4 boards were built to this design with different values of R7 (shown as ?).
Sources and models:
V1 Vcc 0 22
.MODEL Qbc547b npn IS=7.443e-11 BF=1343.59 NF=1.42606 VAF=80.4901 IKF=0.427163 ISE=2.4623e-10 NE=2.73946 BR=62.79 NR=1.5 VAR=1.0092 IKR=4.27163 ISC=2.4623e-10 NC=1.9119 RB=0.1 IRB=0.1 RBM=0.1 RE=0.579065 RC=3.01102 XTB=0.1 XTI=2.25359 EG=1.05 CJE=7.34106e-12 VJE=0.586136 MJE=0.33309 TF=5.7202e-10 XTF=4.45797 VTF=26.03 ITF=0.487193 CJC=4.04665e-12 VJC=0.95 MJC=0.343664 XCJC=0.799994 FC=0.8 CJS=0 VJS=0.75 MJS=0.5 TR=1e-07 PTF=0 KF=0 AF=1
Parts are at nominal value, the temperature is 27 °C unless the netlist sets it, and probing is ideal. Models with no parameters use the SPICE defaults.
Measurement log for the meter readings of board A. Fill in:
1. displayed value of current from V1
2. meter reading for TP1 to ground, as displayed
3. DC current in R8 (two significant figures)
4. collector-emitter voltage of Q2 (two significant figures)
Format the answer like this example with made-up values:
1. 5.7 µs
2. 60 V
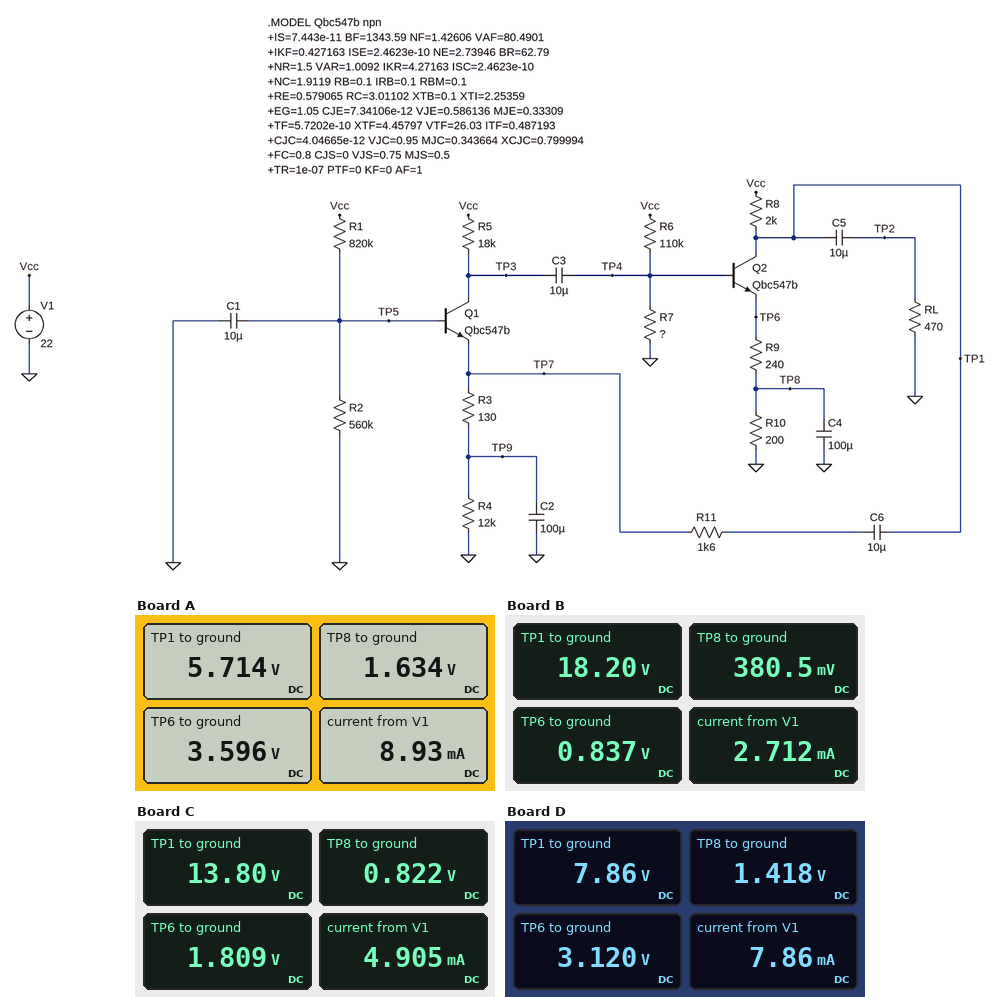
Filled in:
1. 8.93 mA
2. 5.714 V
3. 8.1 mA
4. 2.1 V
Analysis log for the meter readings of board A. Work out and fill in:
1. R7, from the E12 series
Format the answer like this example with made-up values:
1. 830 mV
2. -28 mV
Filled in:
1. 33 kΩ
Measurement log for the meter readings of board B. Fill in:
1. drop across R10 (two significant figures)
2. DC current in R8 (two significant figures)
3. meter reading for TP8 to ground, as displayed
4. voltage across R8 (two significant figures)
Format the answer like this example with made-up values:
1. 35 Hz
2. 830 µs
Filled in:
1. 380 mV
2. 1.9 mA
3. 380.5 mV
4. 3.8 V
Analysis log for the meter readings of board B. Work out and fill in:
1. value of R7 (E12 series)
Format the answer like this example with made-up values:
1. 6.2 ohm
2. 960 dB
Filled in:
1. 8.2 kΩ
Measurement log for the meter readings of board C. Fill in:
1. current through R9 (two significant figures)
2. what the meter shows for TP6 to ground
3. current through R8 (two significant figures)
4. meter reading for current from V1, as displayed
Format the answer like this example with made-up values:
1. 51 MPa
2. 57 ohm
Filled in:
1. 4.1 mA
2. 1.809 V
3. 4.1 mA
4. 4.905 mA
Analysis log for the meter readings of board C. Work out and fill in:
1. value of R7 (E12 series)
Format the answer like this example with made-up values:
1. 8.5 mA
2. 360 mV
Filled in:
1. 15 kΩ
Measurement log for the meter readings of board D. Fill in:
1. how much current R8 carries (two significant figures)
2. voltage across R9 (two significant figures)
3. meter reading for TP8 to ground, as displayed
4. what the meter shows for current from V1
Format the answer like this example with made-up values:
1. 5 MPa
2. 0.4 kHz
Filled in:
1. 7.1 mA
2. 1.7 V
3. 1.418 V
4. 7.86 mA
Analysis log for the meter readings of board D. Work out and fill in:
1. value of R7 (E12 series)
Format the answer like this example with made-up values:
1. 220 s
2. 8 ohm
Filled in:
1. 27 kΩ
